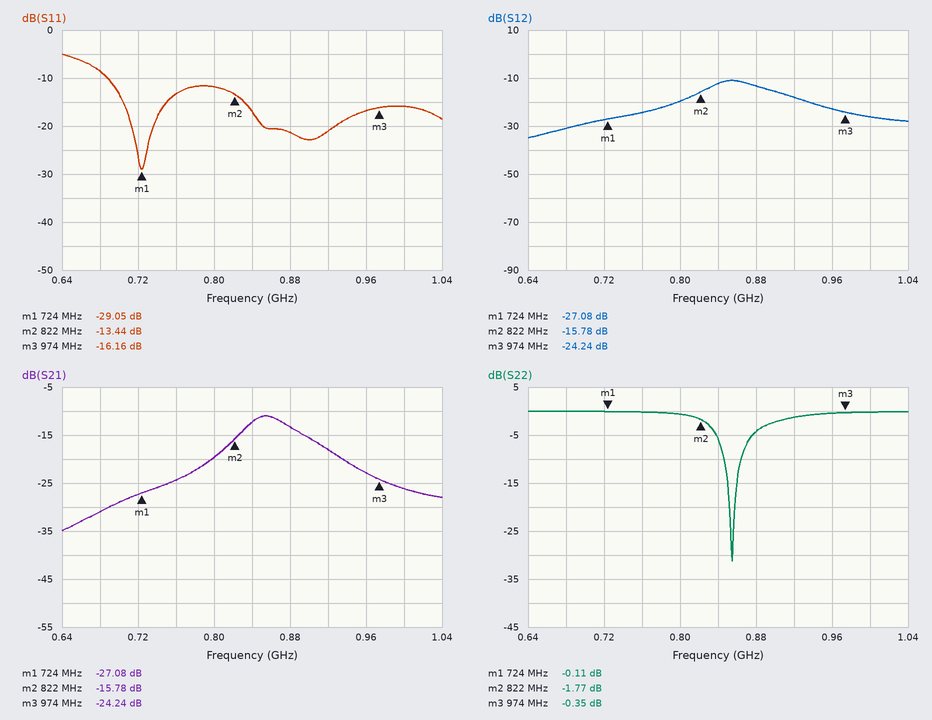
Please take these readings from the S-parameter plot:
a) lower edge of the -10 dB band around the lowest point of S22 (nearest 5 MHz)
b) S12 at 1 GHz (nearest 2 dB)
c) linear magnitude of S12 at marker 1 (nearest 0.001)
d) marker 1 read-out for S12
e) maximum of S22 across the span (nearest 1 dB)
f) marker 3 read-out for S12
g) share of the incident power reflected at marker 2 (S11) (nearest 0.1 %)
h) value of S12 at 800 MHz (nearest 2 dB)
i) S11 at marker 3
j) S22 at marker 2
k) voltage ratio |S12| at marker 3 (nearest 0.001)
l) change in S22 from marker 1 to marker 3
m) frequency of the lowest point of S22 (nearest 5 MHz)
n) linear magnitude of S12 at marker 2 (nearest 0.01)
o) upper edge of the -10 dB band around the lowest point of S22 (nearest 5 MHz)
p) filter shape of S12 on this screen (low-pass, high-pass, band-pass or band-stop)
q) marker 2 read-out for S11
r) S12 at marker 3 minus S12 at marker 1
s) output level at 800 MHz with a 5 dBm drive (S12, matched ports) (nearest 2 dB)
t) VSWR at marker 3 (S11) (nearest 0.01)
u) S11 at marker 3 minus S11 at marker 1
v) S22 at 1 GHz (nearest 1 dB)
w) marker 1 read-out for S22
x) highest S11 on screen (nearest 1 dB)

845 MHz
-26 dB
0.044
-27.08 dB
0 dB
-24.24 dB
4.5 %
-20 dB
-16.16 dB
-1.77 dB
0.061
-0.24 dB
855 MHz
0.16
865 MHz
band-pass
-13.44 dB
2.84 dB
-14 dBm
1.37
12.89 dB
0 dB
-0.11 dB
-5 dB
